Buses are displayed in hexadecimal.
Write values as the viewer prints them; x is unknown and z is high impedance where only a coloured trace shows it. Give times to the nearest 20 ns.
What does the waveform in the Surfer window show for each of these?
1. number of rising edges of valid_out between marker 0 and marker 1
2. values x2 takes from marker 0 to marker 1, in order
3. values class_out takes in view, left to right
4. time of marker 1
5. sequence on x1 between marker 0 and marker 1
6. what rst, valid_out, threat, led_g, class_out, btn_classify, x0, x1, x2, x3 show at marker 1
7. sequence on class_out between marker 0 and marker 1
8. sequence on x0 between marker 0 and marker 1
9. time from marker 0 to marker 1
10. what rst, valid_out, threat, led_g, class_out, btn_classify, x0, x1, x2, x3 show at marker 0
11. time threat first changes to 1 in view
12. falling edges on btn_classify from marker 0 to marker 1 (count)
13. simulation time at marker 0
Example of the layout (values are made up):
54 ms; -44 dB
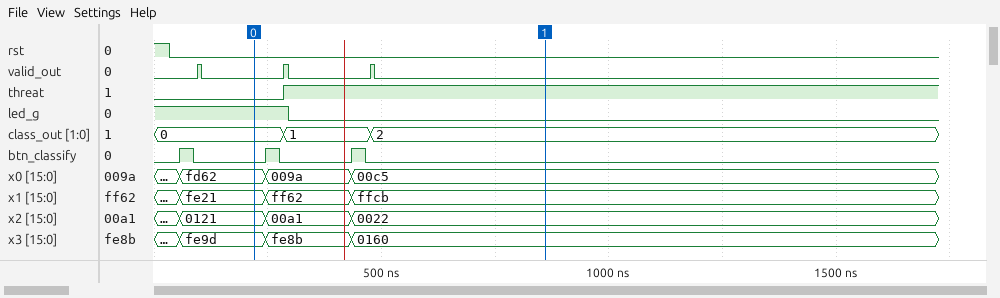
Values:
2; 0121, 00a1, 0022; 0, 1, 2; 860 ns; fe21, ff62, ffcb; rst=0, valid_out=0, threat=1, led_g=0, class_out=2, btn_classify=0, x0=00c5, x1=ffcb, x2=0022, x3=0160; 0, 1, 2; fd62, 009a, 00c5; 640 ns; rst=0, valid_out=0, threat=0, led_g=1, class_out=0, btn_classify=0, x0=fd62, x1=fe21, x2=0121, x3=fe9d; 280 ns; 2; 220 ns
